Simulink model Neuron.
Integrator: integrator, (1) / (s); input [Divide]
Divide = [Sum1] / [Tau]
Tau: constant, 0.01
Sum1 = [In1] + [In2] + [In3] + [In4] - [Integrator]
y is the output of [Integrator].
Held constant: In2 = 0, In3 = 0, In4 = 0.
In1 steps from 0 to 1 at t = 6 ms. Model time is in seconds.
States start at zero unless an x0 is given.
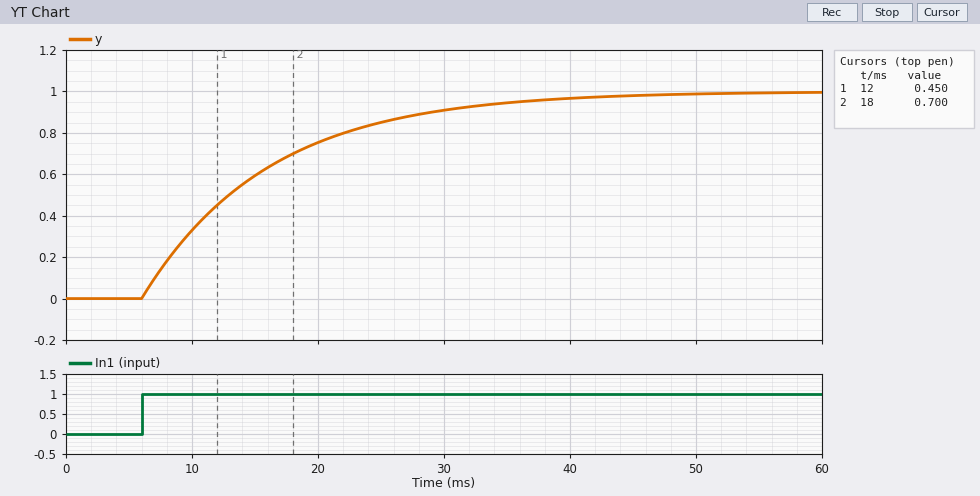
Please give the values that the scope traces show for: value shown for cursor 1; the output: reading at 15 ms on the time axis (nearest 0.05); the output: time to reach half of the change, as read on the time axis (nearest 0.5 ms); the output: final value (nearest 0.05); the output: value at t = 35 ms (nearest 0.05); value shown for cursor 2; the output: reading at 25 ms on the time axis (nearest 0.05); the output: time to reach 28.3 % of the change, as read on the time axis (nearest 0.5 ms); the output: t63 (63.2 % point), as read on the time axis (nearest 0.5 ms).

0.450
0.60
13.0 ms
1.00
0.95
0.700
0.85
9.5 ms
16.0 ms
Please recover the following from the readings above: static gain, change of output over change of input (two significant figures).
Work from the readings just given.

1.0
